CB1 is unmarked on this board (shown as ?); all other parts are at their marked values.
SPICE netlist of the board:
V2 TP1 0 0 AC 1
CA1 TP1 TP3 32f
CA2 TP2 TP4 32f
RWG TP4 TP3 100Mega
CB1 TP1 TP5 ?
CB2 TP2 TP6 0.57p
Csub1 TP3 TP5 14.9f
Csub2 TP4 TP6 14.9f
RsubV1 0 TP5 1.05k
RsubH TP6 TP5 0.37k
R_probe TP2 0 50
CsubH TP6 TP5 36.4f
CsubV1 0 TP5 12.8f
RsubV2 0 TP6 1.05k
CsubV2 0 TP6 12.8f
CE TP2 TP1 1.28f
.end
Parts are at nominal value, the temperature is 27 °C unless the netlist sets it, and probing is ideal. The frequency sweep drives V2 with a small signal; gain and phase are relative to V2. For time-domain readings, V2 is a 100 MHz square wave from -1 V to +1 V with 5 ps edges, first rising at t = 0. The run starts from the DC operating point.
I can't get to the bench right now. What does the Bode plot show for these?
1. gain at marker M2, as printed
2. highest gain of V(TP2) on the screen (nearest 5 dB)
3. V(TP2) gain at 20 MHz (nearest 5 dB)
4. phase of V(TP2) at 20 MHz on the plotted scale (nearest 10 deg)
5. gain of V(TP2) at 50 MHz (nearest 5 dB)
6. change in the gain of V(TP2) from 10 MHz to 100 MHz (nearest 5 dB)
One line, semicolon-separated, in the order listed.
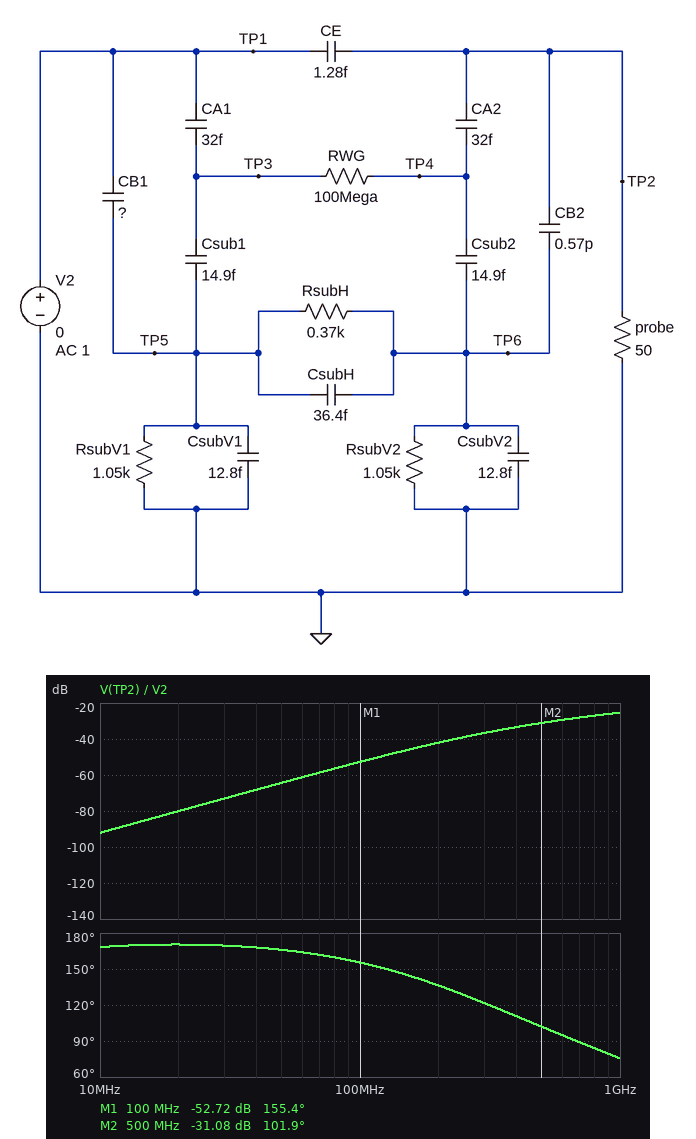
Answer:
-31.08 dB; -25 dB; -80 dB; 170 deg; -65 dB; 40 dB
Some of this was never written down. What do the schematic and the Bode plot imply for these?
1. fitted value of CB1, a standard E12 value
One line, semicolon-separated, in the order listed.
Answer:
470 fF
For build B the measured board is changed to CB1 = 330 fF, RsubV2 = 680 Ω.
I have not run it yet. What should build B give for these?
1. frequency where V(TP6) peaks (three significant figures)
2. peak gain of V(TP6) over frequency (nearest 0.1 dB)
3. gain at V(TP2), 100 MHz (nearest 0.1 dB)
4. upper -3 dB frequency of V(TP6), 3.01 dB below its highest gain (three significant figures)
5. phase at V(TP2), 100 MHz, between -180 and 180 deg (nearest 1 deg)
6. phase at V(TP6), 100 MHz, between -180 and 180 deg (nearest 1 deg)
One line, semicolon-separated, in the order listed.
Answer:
889 MHz; -12.5 dB; -57.8 dB; 3.17 GHz; 161 deg; 74 deg
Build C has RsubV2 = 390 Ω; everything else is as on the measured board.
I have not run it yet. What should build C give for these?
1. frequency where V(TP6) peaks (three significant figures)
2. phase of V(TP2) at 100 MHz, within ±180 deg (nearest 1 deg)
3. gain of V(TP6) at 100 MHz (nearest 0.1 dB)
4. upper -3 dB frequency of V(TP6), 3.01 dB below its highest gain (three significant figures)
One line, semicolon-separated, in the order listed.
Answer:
906 MHz; 163 deg; -23.5 dB; 2.87 GHz
